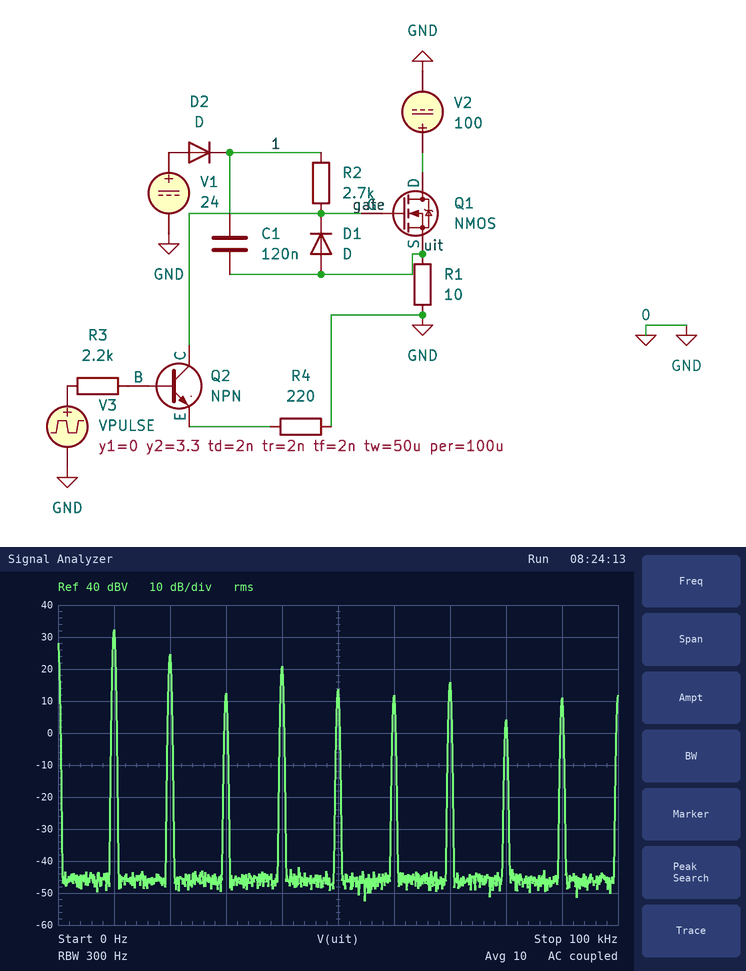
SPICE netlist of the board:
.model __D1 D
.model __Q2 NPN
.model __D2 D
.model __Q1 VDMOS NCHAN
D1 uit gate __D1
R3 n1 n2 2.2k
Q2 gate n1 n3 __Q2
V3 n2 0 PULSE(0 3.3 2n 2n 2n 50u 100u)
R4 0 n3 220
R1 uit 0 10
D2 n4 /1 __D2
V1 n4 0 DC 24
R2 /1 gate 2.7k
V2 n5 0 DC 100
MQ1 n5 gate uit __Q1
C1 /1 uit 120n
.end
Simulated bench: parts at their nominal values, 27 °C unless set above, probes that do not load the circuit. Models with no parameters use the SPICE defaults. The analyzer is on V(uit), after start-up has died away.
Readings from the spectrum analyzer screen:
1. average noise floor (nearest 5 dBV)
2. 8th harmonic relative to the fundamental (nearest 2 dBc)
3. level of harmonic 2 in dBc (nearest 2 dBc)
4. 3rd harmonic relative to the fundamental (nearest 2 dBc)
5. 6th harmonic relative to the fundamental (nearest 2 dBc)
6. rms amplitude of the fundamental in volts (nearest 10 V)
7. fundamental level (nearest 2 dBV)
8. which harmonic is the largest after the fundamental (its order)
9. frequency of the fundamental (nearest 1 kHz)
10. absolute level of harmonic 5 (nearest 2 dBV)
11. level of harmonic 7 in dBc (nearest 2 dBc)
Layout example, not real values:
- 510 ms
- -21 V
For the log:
- -45 dBV
- -28 dBc
- -8 dBc
- -20 dBc
- -20 dBc
- 40 V
- 32 dBV
- 2
- 10 kHz
- 14 dBV
- -16 dBc
